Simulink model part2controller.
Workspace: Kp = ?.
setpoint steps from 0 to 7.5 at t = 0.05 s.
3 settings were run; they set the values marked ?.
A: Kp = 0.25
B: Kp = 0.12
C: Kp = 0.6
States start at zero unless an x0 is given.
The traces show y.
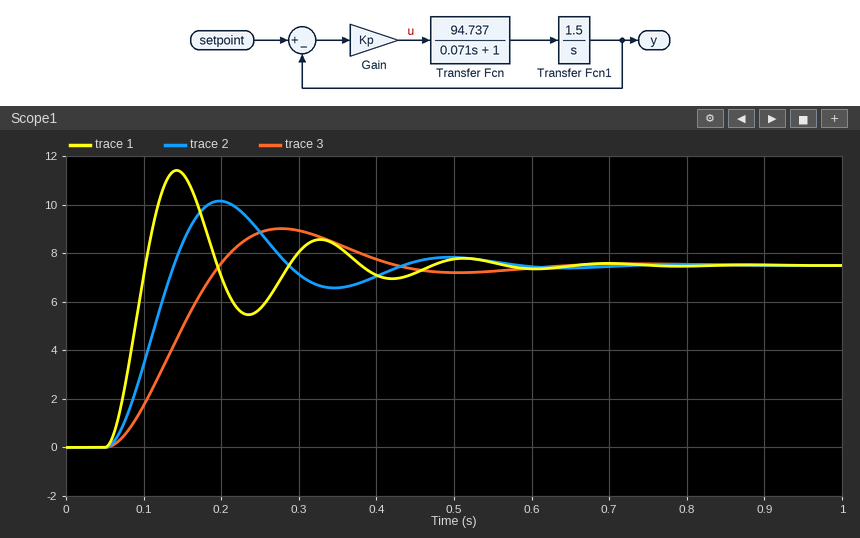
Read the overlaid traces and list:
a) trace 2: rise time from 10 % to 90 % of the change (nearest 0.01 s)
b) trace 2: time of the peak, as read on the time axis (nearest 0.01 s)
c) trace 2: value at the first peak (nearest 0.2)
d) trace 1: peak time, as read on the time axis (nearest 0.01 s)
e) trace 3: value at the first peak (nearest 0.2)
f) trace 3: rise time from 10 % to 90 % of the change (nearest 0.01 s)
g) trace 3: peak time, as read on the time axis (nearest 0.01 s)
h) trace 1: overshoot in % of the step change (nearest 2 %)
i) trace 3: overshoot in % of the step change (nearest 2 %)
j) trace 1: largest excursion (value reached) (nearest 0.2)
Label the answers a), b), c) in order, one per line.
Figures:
a) 0.06 s
b) 0.20 s
c) 10.2
d) 0.14 s
e) 9.0
f) 0.10 s
g) 0.28 s
h) 52 %
i) 20 %
j) 11.4
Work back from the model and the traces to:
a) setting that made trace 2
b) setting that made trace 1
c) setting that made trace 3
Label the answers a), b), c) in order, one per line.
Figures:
a) A
b) C
c) B
